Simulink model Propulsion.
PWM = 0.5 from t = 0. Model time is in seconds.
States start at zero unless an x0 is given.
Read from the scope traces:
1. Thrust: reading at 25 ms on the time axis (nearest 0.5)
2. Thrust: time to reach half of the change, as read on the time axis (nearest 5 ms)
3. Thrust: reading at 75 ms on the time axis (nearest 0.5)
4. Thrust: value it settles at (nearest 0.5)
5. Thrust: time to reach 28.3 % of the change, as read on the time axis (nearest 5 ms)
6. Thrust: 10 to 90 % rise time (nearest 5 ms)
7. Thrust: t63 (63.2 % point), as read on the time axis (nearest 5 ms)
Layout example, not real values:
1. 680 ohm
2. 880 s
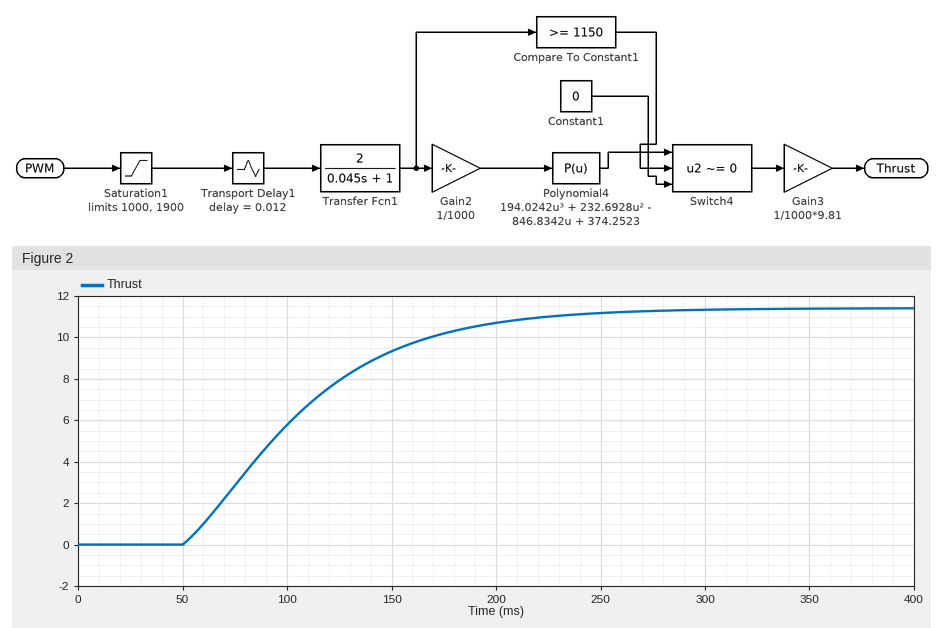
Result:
1. 0.0
2. 100 ms
3. 3.0
4. 11.5
5. 80 ms
6. 115 ms
7. 115 ms
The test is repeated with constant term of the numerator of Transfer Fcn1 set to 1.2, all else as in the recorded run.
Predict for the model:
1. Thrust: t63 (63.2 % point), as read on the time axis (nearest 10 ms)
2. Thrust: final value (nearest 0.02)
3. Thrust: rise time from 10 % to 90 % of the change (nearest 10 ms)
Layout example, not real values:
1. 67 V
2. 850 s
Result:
1. 200 ms
2. 0.28
3. 100 ms
